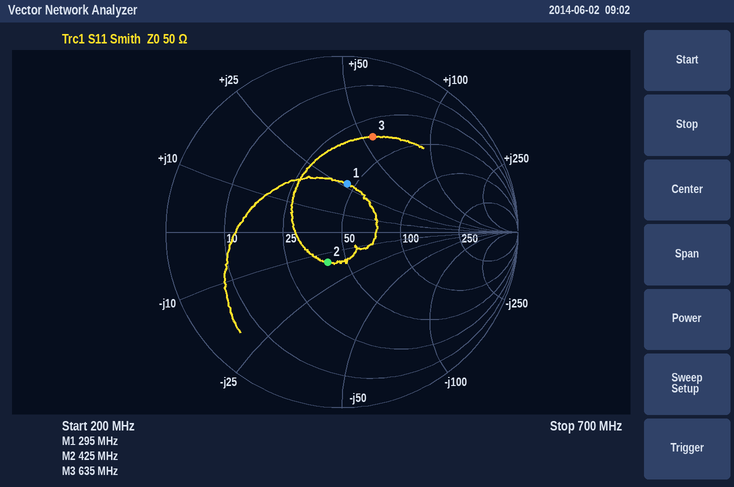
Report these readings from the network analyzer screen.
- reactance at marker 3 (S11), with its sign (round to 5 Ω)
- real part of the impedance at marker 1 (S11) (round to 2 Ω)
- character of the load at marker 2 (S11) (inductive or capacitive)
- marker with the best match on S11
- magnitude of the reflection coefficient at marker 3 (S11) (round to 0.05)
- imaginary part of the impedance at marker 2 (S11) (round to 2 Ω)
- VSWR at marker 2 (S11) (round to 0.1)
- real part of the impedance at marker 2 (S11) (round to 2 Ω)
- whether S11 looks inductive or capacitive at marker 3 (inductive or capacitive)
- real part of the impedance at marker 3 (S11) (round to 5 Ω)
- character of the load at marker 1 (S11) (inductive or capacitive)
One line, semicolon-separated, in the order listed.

+55 Ω; 46 Ω; capacitive; marker 2; 0.55; -14 Ω; 1.5; 40 Ω; inductive; 35 Ω; inductive
